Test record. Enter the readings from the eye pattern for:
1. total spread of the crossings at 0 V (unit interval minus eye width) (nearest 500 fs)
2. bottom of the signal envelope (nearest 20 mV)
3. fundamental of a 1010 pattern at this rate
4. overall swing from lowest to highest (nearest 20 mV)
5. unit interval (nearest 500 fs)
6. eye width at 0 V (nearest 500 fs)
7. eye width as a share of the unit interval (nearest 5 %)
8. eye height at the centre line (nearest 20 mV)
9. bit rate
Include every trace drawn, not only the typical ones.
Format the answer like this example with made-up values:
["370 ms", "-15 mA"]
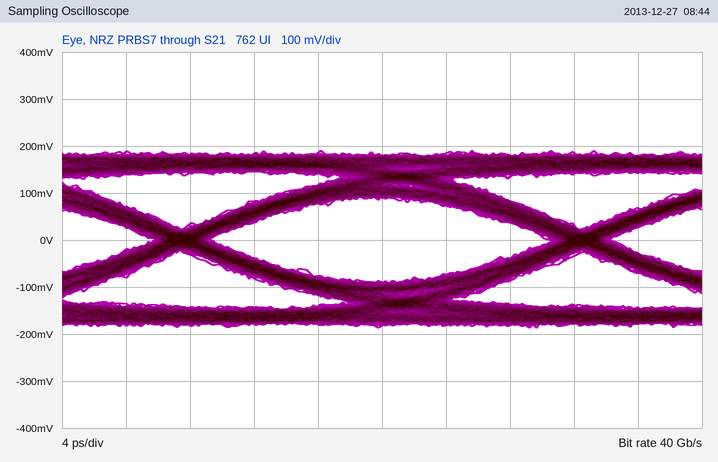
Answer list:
["4.0 ps", "-180 mV", "20 GHz", "380 mV", "25.0 ps", "21.0 ps", "85 %", "180 mV", "40 Gb/s"]
